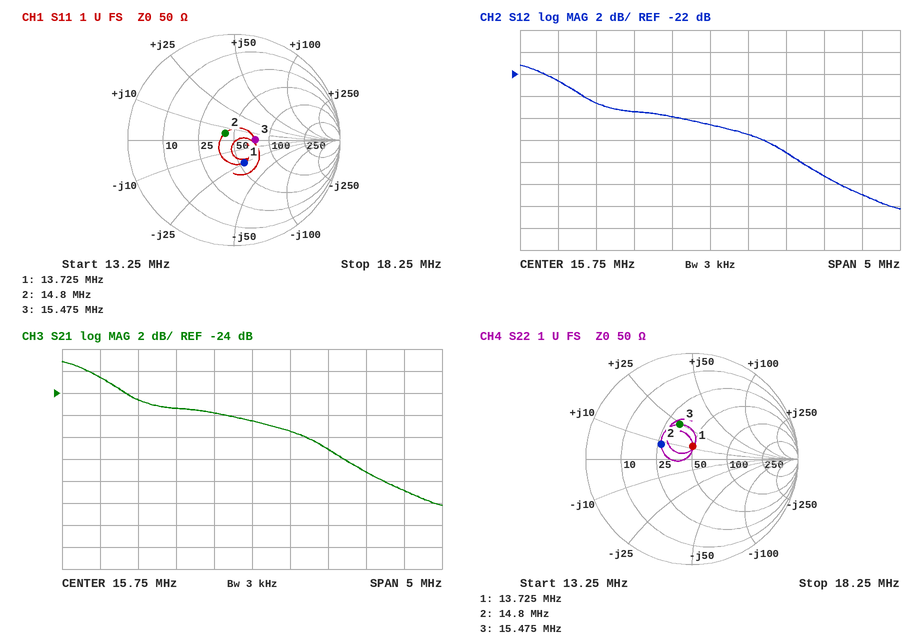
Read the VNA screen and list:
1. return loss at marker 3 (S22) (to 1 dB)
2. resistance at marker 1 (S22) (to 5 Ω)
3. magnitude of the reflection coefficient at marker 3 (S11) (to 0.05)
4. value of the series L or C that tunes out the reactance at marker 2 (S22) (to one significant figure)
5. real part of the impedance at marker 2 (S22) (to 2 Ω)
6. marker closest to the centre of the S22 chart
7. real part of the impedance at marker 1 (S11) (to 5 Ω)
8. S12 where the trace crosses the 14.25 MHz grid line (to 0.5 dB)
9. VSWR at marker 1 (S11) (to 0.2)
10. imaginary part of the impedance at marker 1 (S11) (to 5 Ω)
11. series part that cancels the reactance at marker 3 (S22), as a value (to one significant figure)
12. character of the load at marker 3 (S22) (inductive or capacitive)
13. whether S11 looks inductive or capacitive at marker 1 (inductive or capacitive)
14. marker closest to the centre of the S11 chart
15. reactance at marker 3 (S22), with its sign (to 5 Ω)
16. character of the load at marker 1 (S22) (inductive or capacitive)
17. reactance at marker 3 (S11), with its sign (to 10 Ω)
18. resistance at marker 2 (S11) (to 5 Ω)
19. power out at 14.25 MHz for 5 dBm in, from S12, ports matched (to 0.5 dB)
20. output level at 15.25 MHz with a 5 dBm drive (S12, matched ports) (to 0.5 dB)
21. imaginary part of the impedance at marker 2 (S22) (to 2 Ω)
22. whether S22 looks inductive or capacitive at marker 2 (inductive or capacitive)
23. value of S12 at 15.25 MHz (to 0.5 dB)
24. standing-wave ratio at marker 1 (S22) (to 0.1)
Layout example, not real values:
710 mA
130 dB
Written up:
9 dB
50 Ω
0.20
1 nF
26 Ω
marker 1
55 Ω
-24.5 dB
1.6
-25 Ω
400 pF
inductive
capacitive
marker 2
+25 Ω
inductive
0 Ω
40 Ω
-19.5 dBm
-21.0 dBm
+8 Ω
inductive
-26.0 dB
1.3
